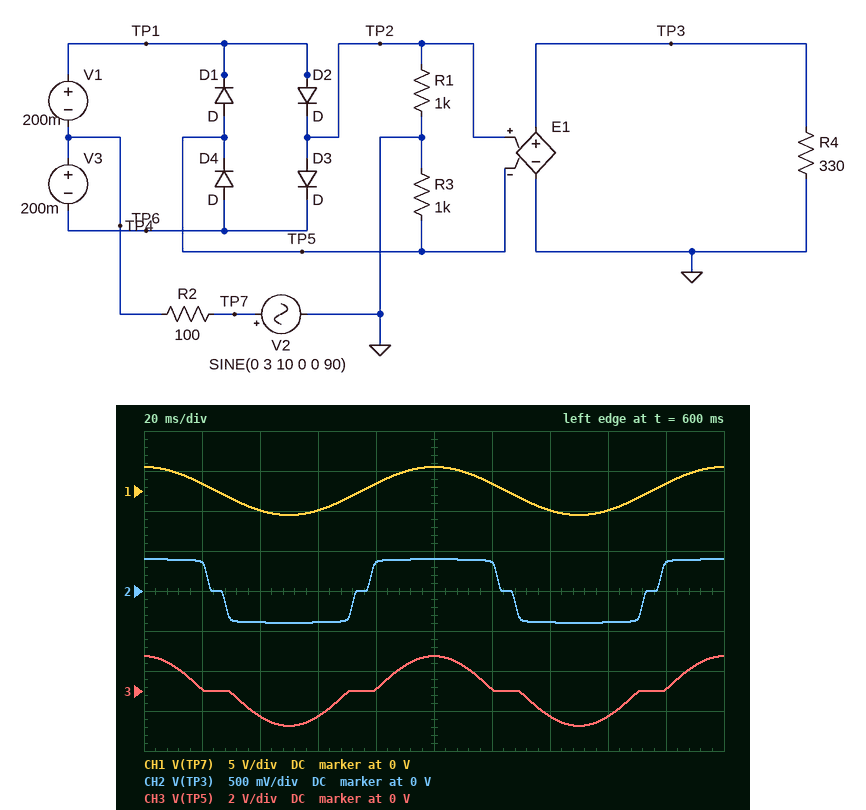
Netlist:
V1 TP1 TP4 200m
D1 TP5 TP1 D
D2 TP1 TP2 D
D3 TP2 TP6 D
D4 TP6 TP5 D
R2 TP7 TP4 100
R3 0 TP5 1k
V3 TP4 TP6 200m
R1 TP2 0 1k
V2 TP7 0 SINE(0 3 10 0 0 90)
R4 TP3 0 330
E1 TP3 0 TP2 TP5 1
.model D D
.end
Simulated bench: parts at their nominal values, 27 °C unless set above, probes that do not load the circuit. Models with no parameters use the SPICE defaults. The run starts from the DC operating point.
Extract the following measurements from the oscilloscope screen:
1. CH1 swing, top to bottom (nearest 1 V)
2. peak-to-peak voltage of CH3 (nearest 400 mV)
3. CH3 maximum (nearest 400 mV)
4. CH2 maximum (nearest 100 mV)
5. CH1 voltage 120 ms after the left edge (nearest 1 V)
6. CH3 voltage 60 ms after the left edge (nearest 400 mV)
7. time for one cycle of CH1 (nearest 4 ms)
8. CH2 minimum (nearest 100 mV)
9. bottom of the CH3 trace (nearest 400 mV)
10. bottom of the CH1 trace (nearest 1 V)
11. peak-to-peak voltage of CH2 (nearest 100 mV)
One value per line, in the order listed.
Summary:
6 V
3.6 V
1.6 V
400 mV
1 V
-1.2 V
100 ms
-400 mV
-1.6 V
-3 V
800 mV
